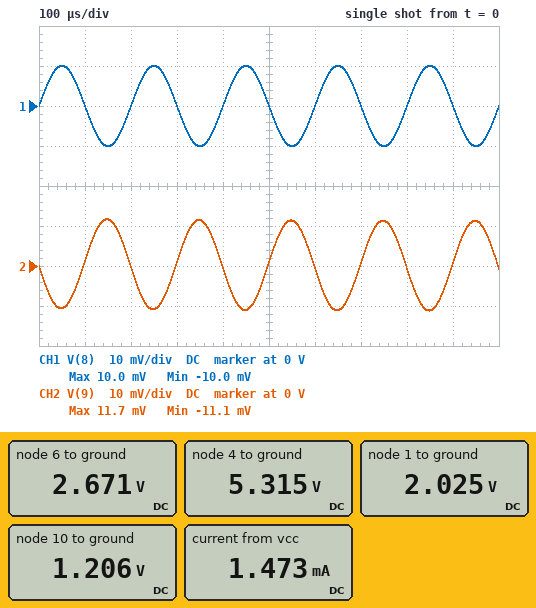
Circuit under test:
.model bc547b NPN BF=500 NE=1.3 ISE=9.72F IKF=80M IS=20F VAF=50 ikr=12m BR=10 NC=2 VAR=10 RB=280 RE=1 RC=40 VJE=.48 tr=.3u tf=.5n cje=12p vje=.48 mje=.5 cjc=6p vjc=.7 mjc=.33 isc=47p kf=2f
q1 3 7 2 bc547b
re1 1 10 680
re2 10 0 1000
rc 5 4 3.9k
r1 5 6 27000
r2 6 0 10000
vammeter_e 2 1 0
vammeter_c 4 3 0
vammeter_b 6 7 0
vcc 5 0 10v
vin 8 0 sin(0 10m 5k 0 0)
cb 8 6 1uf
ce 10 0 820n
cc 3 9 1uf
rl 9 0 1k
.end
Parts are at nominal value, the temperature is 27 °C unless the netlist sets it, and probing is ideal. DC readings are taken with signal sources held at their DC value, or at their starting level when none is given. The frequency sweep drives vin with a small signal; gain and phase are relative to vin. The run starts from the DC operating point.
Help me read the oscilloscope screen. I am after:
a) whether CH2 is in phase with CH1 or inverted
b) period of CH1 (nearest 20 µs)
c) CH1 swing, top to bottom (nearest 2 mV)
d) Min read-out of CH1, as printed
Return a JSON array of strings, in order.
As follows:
["inverted", "200 µs", "20 mV", "-10.0 mV"]
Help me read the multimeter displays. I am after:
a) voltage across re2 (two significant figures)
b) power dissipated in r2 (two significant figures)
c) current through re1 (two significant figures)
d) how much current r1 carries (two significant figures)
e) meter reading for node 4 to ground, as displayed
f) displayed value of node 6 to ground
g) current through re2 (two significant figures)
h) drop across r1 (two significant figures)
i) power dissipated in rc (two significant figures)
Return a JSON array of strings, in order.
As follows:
["1.2 V", "710 µW", "1.2 mA", "270 µA", "5.315 V", "2.671 V", "1.2 mA", "7.3 V", "5.6 mW"]
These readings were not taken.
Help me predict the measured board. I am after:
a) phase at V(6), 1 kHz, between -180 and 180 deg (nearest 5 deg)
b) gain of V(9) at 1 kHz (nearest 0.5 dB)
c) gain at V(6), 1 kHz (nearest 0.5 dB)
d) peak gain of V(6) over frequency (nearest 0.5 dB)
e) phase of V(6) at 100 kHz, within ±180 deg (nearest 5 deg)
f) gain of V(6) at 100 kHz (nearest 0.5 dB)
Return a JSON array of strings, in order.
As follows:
["0 deg", "0.5 dB", "0 dB", "0 dB", "0 deg", "0 dB"]
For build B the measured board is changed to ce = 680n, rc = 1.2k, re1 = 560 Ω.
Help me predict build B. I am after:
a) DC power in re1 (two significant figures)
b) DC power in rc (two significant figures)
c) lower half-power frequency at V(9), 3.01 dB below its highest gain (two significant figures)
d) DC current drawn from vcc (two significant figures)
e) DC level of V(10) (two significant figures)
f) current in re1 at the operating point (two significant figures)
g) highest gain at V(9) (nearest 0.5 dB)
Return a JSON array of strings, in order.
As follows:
["940 µW", "2.0 mW", "560 Hz", "1.6 mA", "1.3 V", "1.3 mA", "-0.5 dB"]
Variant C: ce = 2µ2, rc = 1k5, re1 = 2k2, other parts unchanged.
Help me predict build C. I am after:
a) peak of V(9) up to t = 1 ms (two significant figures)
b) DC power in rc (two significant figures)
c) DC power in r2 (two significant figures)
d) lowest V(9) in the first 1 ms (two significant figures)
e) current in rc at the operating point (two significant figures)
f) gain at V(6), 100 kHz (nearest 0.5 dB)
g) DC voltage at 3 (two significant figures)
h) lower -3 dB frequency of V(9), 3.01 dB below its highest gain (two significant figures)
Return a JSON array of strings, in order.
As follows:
["2.7 mV", "620 µW", "720 µW", "-2.6 mV", "640 µA", "0 dB", "9.0 V", "35 MHz"]
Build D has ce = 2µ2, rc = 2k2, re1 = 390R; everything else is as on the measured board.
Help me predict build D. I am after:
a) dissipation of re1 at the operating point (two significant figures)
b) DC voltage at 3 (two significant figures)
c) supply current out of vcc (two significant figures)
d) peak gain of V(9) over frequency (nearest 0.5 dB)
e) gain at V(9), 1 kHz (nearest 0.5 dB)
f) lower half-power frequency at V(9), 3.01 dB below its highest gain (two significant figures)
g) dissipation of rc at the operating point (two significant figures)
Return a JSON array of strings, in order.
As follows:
["820 µW", "6.8 V", "1.7 mA", "4.5 dB", "4.0 dB", "240 Hz", "4.6 mW"]
